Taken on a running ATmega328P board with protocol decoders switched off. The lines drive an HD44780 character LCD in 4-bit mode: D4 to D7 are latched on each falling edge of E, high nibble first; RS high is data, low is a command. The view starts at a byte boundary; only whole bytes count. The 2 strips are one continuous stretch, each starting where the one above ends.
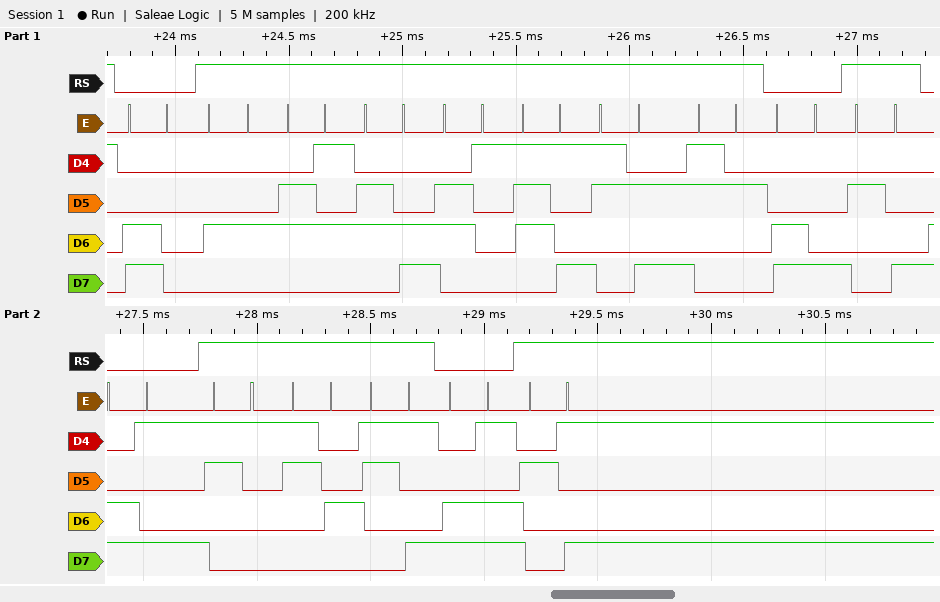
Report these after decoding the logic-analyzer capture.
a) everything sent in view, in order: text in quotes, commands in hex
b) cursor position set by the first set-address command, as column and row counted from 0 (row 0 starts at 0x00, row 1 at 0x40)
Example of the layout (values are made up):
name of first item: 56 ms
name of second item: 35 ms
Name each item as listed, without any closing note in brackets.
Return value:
everything sent in view, in order: text in quotes, commands in hex: 0xC0 "Delay:2" 0xC8 "(" 0xC9 "149" 0xCD ")"
cursor position set by the first set-address command, as column and row counted from 0: column 0, row 1
